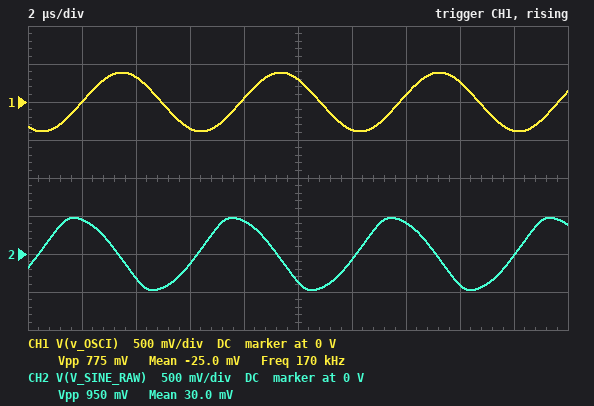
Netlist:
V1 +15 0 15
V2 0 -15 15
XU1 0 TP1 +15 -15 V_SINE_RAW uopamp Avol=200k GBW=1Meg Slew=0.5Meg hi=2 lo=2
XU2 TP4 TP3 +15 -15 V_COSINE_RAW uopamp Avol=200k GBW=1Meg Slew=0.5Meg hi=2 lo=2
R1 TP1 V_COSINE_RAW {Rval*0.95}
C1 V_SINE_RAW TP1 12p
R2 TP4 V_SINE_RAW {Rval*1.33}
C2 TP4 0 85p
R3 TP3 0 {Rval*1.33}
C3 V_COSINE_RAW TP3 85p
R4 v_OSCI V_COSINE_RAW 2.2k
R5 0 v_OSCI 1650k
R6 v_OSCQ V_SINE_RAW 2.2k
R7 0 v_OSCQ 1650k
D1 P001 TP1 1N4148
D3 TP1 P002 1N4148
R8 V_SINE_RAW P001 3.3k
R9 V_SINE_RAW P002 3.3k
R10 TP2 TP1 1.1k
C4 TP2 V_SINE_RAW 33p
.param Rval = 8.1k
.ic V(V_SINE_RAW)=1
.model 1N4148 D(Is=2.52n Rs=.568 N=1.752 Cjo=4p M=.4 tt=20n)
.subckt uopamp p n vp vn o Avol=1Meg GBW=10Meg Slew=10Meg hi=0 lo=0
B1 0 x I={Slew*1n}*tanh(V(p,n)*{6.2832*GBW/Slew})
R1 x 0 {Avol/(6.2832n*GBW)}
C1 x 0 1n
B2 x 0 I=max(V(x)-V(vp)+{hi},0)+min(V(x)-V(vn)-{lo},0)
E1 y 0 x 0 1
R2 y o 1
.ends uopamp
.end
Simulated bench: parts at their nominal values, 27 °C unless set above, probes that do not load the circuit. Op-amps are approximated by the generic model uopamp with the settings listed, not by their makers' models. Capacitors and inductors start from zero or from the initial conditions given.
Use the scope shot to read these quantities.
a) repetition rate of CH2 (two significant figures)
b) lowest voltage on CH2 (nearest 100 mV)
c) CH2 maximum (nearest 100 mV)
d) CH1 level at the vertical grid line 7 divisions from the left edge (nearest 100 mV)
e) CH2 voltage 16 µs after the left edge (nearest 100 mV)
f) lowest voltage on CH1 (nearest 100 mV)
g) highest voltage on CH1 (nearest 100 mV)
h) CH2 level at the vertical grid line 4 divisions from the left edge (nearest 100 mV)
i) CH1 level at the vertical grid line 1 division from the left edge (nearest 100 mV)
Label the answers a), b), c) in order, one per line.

a) 170 kHz
b) -500 mV
c) 500 mV
d) 100 mV
e) -400 mV
f) -400 mV
g) 400 mV
h) 400 mV
i) 0 V
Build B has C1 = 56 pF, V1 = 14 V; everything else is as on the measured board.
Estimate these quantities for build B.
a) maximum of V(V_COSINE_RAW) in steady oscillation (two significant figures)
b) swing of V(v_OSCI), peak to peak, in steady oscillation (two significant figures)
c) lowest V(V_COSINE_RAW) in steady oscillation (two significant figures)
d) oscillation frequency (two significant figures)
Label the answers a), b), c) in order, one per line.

a) 490 mV
b) 980 mV
c) -490 mV
d) 140 kHz
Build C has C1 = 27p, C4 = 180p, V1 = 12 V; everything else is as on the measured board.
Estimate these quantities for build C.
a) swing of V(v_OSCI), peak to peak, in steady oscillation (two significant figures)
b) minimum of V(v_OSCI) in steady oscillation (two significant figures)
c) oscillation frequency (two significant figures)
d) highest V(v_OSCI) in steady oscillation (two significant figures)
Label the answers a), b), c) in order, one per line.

a) 1.1 V
b) -570 mV
c) 110 kHz
d) 570 mV
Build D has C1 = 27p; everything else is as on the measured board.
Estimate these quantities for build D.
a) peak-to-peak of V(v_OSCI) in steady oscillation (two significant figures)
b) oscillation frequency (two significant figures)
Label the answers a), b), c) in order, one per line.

a) 850 mV
b) 160 kHz
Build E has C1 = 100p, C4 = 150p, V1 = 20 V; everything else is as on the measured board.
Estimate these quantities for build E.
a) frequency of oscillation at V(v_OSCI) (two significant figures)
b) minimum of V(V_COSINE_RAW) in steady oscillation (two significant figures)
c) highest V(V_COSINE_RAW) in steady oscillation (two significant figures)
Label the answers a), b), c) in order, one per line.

a) 100 kHz
b) -680 mV
c) 680 mV
